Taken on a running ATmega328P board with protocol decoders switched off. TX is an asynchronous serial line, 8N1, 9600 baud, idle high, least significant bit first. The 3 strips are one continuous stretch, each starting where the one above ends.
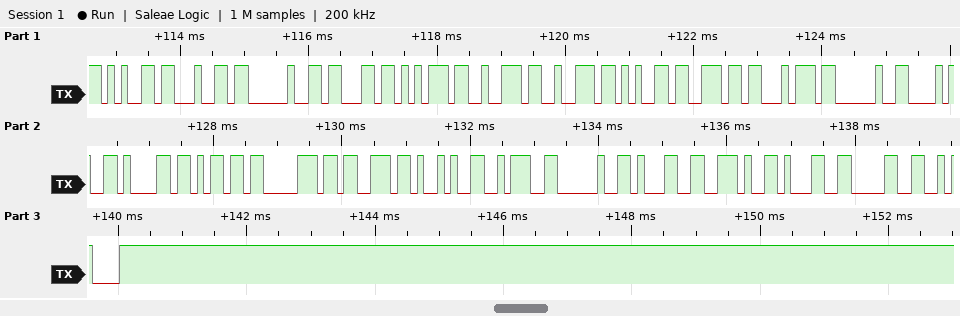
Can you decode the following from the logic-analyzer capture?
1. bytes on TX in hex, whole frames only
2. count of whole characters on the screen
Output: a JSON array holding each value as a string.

["65 64 20 63 75 72 72 65 6E 74 20 28 61 6D 70 73 29 3A 20 31 2E 31 30 0A", "24"]
